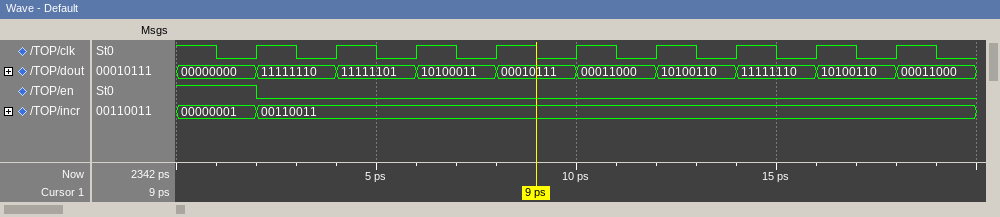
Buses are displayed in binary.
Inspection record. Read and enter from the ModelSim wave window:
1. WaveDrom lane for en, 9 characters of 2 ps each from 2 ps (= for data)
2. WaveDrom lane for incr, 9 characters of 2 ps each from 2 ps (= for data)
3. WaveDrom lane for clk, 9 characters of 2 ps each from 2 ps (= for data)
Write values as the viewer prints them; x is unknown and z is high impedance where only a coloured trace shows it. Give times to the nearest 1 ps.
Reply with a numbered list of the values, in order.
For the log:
1. {name: 'en', wave: '0........'}
2. {name: 'incr', wave: '=........', data: '00110011'}
3. {name: 'clk', wave: 'p........'}
